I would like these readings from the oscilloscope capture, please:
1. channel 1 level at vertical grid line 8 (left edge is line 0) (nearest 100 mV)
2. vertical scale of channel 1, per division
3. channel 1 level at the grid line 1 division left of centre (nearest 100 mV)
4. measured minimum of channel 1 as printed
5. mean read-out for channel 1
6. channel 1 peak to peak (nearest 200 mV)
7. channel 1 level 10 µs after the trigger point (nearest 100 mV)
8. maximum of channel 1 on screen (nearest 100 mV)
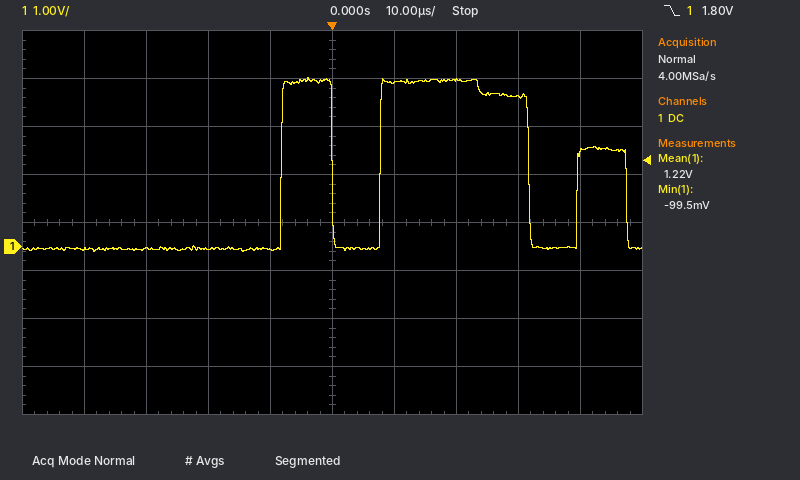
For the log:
3.1 V
1 V
-100 mV
-99.5 mV
1.22 V
3.6 V
3.4 V
3.5 V
